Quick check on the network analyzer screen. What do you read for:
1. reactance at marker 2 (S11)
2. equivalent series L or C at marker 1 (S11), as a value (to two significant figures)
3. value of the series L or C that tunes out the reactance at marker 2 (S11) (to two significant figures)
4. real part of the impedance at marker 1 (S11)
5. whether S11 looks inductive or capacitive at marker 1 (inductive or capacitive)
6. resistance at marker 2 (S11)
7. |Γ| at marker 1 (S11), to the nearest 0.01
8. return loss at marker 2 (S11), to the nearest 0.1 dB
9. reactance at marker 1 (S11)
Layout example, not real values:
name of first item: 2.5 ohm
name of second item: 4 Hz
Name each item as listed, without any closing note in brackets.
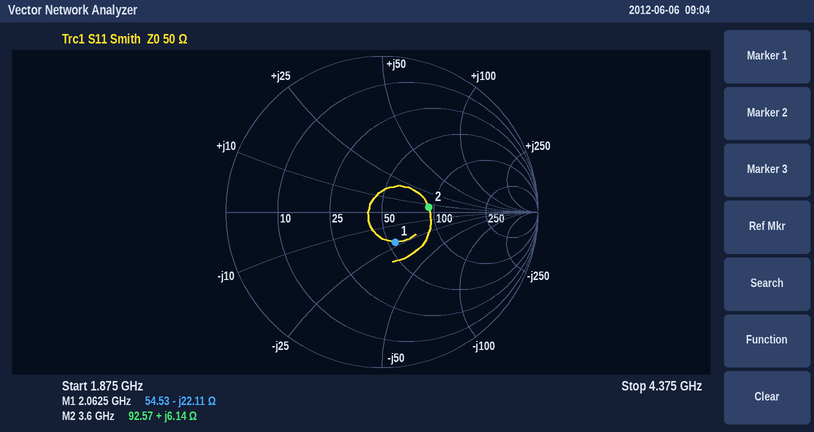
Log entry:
reactance at marker 2: +6.14 Ω
equivalent series L or C at marker 1 (S11), as a value: 3.5 pF
value of the series L or C that tunes out the reactance at marker 2 (S11): 7.2 pF
real part of the impedance at marker 1: 54.53 Ω
whether S11 looks inductive or capacitive at marker 1: capacitive
resistance at marker 2: 92.57 Ω
|Γ| at marker 1 (S11), to the nearest 0.01: 0.21
return loss at marker 2 (S11), to the nearest 0.1 dB: 10.4 dB
reactance at marker 1: -22.11 Ω
